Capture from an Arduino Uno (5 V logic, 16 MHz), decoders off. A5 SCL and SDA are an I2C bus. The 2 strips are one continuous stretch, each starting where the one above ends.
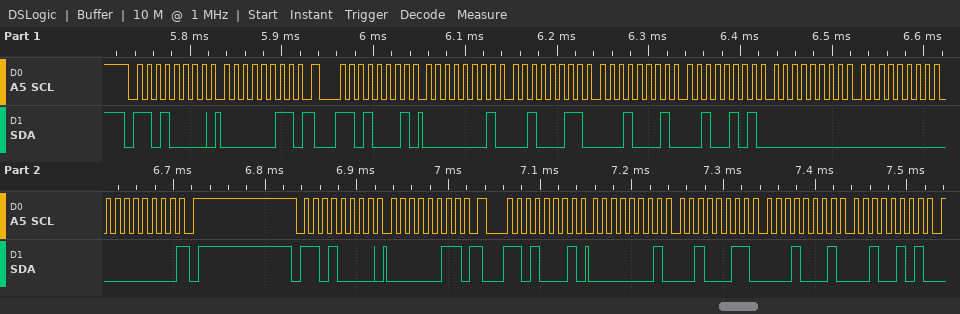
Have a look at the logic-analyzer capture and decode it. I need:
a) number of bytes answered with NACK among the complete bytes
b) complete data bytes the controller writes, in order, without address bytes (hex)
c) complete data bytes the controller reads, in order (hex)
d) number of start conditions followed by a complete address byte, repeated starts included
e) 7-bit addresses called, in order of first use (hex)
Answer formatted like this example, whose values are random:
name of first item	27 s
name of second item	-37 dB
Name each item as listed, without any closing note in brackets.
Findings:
number of bytes answered with NACK among the complete bytes	1
complete data bytes the controller writes, in order, without address bytes	03 03
complete data bytes the controller reads, in order	01 23 11 25 00 00 00 01 23 11 25
number of start conditions followed by a complete address byte, repeated starts included	4
7-bit addresses called, in order of first use	0x68
